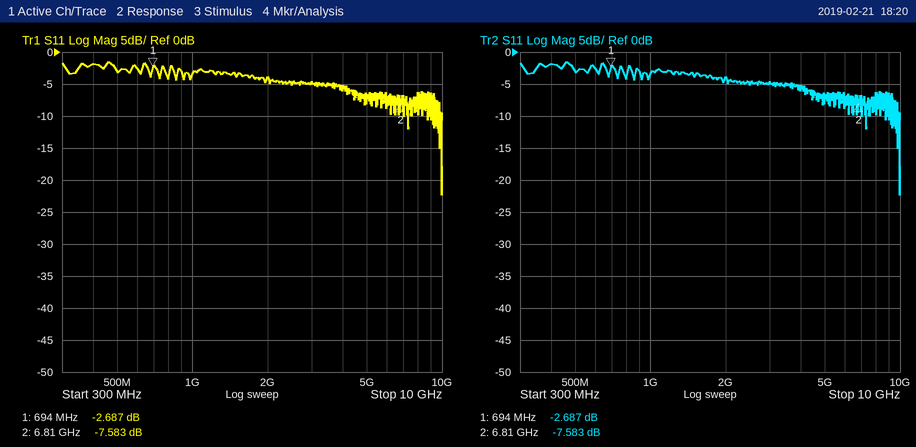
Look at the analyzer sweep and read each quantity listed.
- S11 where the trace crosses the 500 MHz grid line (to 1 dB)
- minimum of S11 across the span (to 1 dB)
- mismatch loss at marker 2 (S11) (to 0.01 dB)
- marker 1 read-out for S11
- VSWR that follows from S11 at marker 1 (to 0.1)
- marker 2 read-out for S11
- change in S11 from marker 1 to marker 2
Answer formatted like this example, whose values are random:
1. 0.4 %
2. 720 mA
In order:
1. -3 dB
2. -22 dB
3. 0.83 dB
4. -2.687 dB
5. 6.5
6. -7.583 dB
7. -4.896 dB
